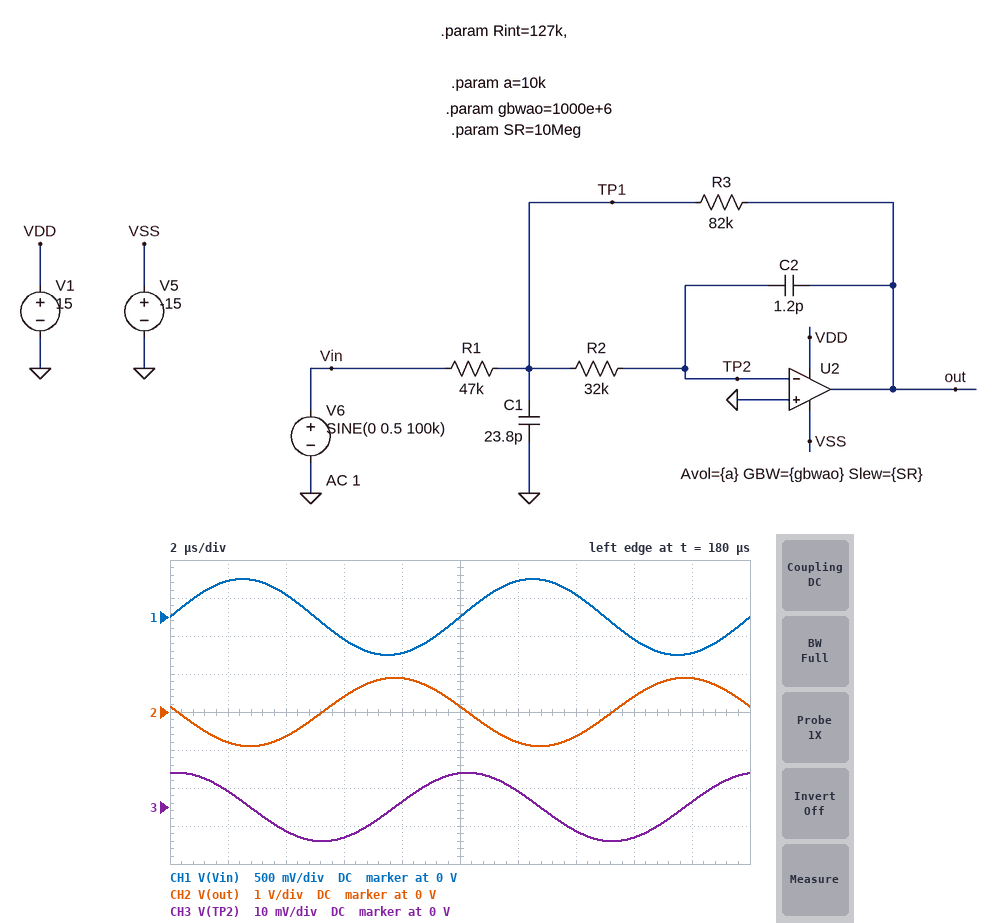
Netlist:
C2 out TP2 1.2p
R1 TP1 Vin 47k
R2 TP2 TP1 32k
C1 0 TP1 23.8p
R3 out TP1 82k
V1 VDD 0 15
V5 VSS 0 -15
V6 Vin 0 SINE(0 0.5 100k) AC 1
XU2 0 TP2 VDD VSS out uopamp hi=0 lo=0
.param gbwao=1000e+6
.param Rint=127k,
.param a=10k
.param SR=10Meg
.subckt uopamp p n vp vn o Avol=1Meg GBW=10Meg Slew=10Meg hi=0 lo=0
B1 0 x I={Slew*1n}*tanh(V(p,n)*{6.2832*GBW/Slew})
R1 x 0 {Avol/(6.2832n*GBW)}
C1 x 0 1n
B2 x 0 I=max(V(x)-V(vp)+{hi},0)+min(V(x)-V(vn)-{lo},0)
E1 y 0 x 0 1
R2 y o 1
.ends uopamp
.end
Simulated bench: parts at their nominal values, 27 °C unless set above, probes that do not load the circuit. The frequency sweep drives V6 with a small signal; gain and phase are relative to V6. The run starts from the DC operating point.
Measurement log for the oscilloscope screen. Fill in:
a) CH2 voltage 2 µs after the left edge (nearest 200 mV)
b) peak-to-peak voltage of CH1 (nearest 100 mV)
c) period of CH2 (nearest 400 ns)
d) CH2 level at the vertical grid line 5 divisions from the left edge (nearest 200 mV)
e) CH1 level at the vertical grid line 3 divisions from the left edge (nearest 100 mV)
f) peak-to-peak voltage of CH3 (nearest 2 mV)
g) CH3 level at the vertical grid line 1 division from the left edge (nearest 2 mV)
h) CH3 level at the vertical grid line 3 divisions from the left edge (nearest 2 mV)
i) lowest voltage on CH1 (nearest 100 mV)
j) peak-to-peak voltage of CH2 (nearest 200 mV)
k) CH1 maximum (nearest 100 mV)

-800 mV
1.0 V
10.0 µs
200 mV
-300 mV
18 mV
4 mV
-8 mV
-500 mV
1.8 V
500 mV
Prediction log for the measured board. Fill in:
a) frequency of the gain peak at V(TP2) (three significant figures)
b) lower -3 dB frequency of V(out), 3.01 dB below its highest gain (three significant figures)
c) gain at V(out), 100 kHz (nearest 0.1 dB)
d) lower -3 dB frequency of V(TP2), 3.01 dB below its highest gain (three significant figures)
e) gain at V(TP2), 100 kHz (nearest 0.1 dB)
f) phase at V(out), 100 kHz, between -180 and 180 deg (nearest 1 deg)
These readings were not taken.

487 kHz
122 kHz
5.1 dB
342 kHz
-34.9 dB
171 deg
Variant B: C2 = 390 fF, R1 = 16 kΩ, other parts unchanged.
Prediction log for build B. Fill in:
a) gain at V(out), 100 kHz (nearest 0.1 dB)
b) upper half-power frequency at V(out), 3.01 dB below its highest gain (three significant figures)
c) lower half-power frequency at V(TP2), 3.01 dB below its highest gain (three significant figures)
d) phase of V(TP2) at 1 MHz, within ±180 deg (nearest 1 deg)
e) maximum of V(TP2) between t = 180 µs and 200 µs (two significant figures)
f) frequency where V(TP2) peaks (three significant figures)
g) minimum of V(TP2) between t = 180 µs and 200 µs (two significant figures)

14.3 dB
800 kHz
447 kHz
-46 deg
26 mV
674 kHz
-26 mV
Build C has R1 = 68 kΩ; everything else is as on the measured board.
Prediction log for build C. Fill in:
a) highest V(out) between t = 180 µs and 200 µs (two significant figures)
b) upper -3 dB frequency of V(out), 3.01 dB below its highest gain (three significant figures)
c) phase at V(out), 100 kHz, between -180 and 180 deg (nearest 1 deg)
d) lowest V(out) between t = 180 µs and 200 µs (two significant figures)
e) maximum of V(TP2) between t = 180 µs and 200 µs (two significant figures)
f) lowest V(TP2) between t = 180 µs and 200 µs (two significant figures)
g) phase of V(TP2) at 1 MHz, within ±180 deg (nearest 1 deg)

620 mV
577 kHz
172 deg
-620 mV
6.2 mV
-6.2 mV
-72 deg
